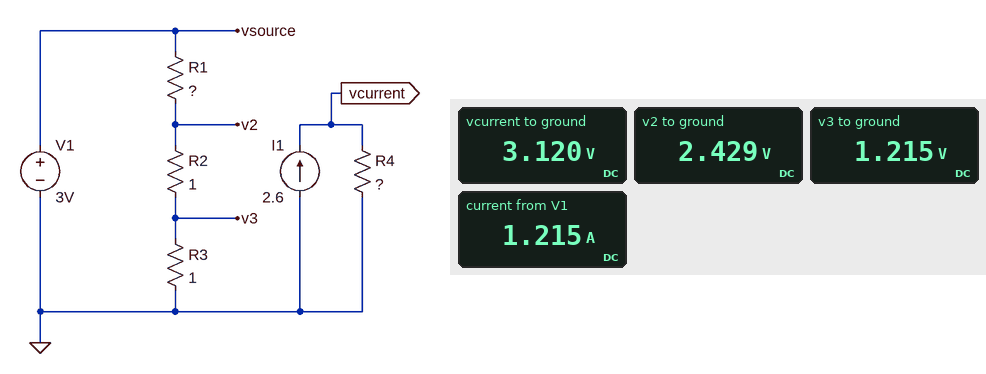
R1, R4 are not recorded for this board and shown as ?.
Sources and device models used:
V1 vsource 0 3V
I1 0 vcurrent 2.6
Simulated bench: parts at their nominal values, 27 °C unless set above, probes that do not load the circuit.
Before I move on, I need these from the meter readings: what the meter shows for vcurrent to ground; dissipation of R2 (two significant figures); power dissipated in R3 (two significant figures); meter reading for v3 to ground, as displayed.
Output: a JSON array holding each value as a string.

["3.120 V", "1.5 W", "1.5 W", "1.215 V"]
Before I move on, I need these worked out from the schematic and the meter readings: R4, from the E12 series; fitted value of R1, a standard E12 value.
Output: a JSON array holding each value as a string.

["1.2 Ω", "0.47 Ω"]
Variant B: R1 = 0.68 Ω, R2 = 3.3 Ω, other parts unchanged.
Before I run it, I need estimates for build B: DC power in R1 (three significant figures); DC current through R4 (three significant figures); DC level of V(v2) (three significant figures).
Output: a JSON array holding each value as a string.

["247 mW", "2.60 A", "2.59 V"]
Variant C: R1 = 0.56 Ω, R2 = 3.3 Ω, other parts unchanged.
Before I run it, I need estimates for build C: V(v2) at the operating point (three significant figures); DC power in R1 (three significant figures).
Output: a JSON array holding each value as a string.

["2.65 V", "213 mW"]
